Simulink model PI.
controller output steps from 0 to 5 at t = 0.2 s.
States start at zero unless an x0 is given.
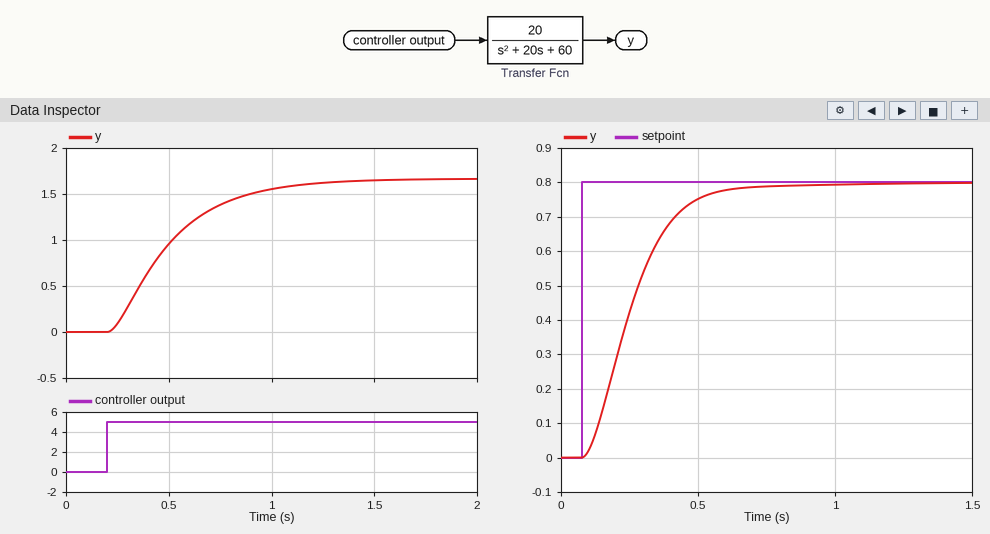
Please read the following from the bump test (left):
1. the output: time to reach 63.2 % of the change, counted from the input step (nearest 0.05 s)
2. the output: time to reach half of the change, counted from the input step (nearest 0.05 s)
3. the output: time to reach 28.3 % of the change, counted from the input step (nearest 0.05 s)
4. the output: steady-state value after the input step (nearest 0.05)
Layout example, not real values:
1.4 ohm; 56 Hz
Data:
0.35 s; 0.25 s; 0.15 s; 1.65
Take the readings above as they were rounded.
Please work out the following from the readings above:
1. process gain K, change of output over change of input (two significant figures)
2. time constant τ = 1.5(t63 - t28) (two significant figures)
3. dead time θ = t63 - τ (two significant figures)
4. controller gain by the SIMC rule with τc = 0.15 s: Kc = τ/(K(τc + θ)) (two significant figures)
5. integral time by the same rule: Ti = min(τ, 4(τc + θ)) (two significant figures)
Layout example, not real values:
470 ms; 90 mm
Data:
0.33; 0.30 s; 0.050 s; 4.5; 0.30 s
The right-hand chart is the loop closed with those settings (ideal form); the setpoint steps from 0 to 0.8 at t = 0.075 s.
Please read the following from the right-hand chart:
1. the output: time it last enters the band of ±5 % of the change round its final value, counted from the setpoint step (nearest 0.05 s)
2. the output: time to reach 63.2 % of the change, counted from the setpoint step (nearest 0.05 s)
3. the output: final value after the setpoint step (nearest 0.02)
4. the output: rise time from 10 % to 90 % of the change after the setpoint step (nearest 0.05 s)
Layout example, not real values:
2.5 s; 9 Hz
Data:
0.45 s; 0.20 s; 0.80; 0.30 s
